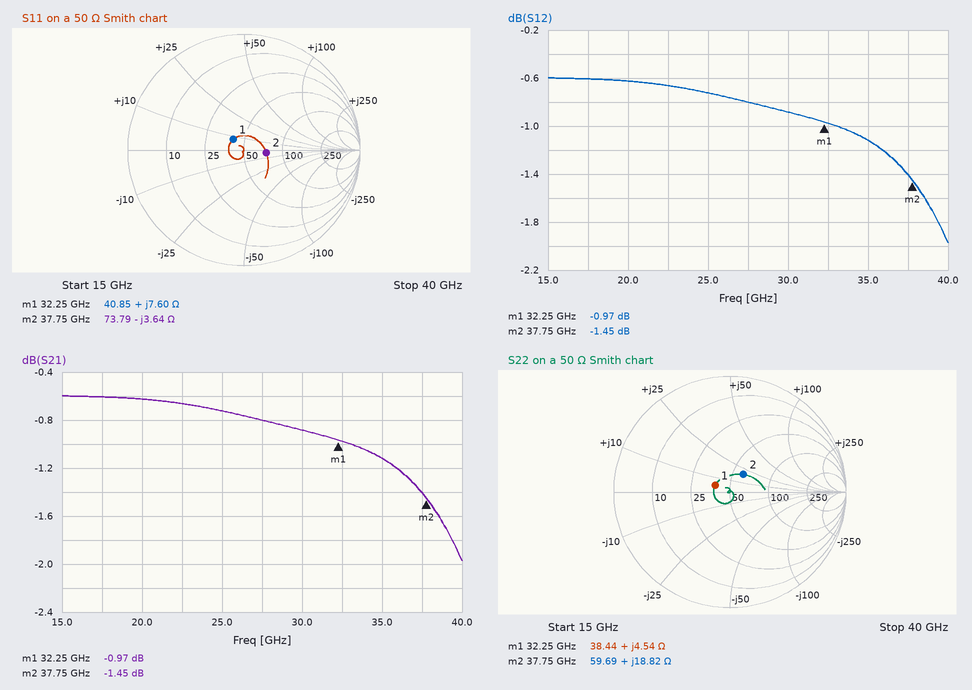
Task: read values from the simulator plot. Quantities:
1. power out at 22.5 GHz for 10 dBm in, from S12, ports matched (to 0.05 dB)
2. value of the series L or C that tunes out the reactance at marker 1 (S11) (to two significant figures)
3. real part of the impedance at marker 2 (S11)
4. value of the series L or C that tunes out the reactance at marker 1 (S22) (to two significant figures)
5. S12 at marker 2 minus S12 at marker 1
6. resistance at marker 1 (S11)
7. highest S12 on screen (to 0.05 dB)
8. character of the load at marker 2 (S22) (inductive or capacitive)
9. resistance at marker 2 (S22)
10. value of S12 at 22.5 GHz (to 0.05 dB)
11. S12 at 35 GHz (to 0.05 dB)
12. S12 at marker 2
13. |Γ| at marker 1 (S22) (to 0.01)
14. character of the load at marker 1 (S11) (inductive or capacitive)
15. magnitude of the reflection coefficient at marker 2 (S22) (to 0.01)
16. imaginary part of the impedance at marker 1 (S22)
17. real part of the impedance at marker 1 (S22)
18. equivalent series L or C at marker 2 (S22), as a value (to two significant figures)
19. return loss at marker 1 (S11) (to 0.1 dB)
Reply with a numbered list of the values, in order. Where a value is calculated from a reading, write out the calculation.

1. 10 dBm + (-0.65 dB) = 9.35 dBm
2. C = 1/(2π × 32.25 GHz × 7.6 Ω) ≈ 649 fF, so 650 fF to two significant figures
3. 73.79 Ω
4. C = 1/(2π × 32.25 GHz × 4.54 Ω) ≈ 1.1 pF
5. -1.45 − (-0.97) = -0.48 dB
6. 40.85 Ω
7. -0.60 dB
8. inductive
9. 59.69 Ω
10. -0.65 dB
11. -1.10 dB
12. -1.45 dB
13. 0.14
14. inductive
15. 0.19
16. +4.54 Ω
17. 38.44 Ω
18. L = 18.82 Ω/(2π × 37.75 GHz) ≈ 79 pH
19. 17.7 dB
